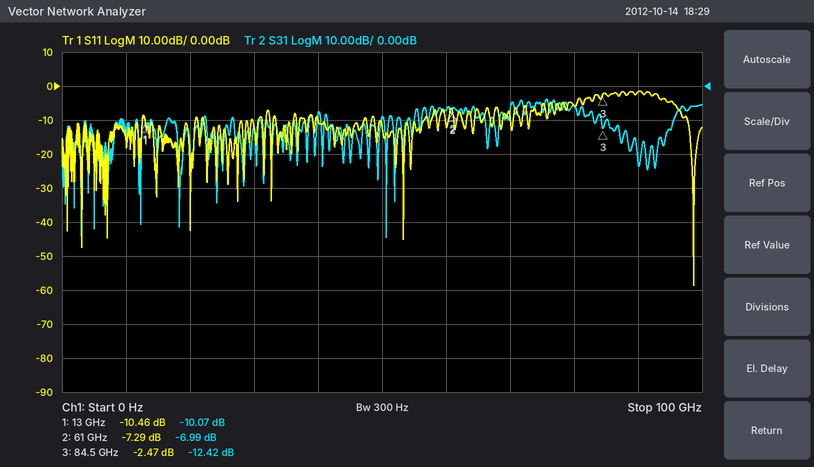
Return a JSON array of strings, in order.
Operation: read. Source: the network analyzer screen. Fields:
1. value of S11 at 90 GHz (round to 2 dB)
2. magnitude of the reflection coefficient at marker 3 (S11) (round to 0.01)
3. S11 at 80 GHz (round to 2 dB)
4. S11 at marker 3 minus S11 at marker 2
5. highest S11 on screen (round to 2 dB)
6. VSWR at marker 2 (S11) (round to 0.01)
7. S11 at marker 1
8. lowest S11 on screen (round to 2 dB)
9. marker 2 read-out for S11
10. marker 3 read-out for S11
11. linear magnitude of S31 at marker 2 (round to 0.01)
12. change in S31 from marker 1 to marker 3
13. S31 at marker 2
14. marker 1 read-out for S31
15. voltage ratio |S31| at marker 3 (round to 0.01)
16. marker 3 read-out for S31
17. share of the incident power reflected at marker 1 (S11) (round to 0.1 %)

["-2 dB", "0.75", "-6 dB", "4.82 dB", "-2 dB", "2.52", "-10.46 dB", "-58 dB", "-7.29 dB", "-2.47 dB", "0.45", "-2.35 dB", "-6.99 dB", "-10.07 dB", "0.24", "-12.42 dB", "9.0 %"]
